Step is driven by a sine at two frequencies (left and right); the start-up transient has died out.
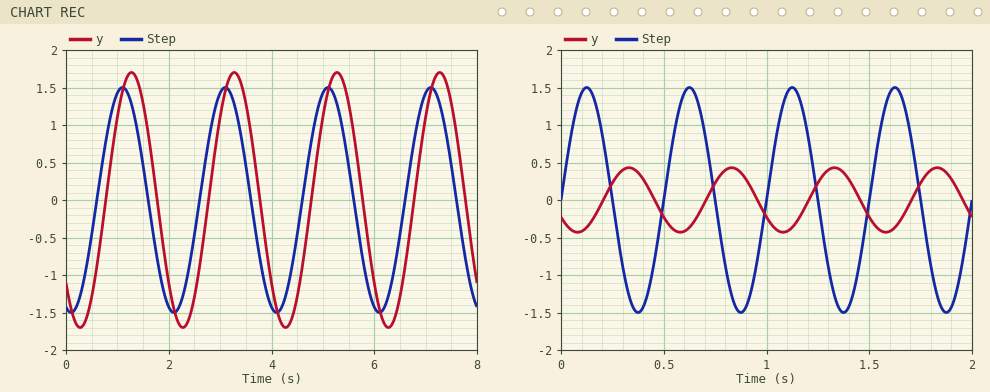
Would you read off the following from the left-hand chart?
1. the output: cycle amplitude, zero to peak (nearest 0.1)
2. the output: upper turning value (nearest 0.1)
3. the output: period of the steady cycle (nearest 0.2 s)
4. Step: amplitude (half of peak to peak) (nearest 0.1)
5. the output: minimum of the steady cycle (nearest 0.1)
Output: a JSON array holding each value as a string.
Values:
["1.7", "1.7", "2.0 s", "1.5", "-1.7"]
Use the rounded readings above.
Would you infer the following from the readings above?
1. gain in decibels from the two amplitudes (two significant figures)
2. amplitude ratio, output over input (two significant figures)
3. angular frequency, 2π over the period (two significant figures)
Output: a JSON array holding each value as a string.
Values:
["1.1 dB", "1.1", "3.1 rad/s"]
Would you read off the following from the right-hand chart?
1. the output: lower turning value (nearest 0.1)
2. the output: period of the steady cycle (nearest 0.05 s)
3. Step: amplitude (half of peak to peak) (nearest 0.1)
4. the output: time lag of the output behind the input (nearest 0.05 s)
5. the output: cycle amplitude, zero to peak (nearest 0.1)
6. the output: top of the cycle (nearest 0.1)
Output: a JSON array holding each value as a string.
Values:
["-0.4", "0.50 s", "1.5", "0.20 s", "0.4", "0.4"]
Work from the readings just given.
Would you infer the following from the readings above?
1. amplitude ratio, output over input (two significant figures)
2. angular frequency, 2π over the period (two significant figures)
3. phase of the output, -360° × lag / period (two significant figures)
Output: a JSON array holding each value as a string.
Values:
["0.27", "13 rad/s", "-140°"]
